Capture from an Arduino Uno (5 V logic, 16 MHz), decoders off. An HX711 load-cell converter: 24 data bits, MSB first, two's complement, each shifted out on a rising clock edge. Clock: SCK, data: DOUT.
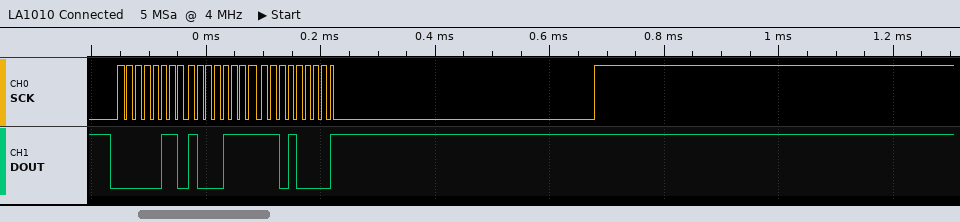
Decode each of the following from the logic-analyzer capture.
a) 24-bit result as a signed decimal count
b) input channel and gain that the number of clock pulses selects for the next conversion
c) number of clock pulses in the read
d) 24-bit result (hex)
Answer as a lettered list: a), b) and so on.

a) 430032
b) channel B, gain 32
c) 26
d) 0x068FD0
